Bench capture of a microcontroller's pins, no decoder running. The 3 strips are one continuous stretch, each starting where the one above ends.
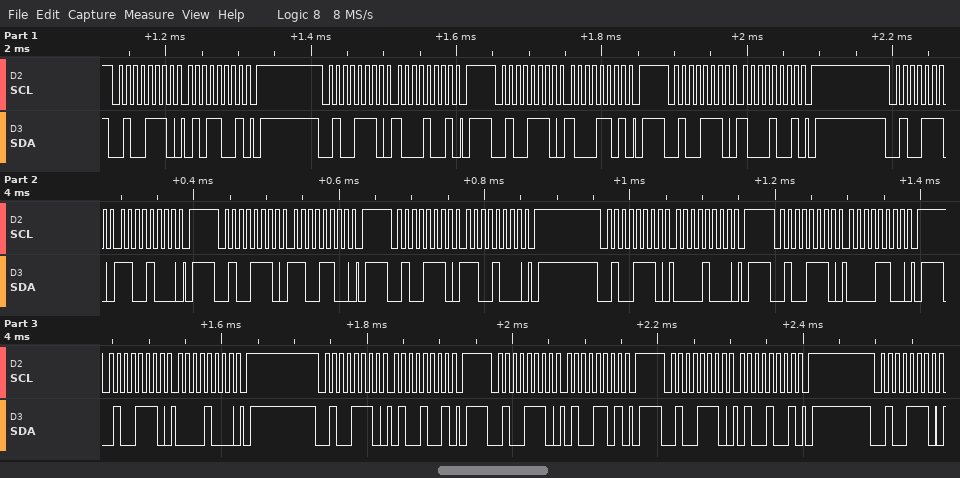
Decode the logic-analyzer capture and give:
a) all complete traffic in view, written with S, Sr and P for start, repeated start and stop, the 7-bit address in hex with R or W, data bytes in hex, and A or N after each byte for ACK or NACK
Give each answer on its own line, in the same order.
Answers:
S 27W A 59 A P S 27W A 89 A P S 27W A 8D A P S 27W A 89 A P S 27W A C8 A P S 27W A CC A P S 27W A C8 A P S 27W A 08 A P S 27W A 0C A P S 27W A 08 A P S 27W A 49 A P S 27W A 4D A P S 27W A 49 A P S 27W A
